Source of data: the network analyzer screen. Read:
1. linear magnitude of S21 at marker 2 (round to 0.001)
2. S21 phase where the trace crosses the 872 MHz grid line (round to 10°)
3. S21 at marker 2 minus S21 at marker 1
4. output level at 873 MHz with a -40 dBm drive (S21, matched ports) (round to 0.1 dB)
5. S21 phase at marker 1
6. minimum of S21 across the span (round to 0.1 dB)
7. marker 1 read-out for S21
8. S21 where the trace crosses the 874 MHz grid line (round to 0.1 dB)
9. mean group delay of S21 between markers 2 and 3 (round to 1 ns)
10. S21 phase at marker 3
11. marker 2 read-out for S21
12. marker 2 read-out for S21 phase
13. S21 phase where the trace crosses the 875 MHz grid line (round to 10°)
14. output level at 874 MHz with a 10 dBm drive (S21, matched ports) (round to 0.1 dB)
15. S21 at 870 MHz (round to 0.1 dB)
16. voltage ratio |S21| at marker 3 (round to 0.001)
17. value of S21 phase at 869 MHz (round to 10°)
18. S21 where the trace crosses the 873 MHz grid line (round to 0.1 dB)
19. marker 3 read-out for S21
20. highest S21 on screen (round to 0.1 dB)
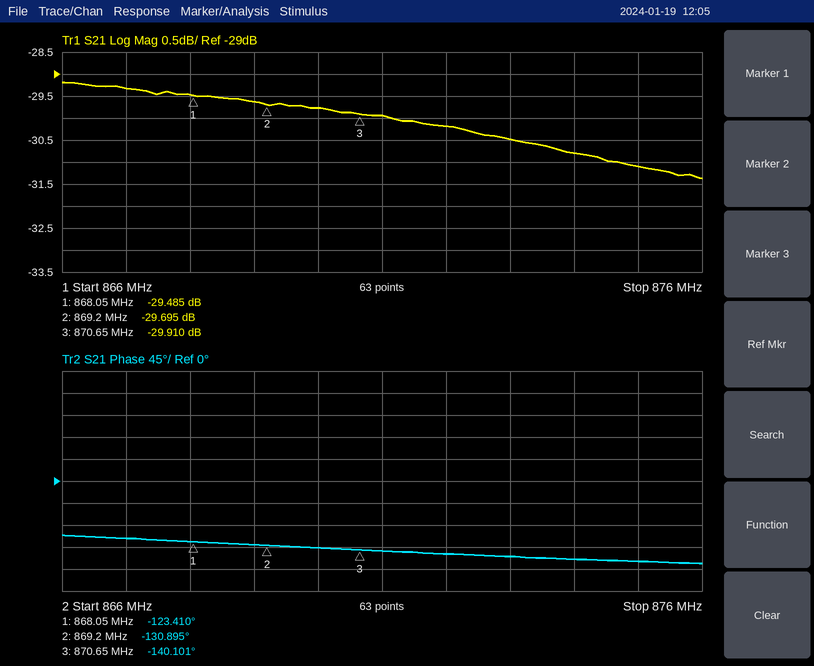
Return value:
0.033
-150°
-0.210 dB
-70.5 dBm
-123.410°
-31.4 dB
-29.485 dB
-30.8 dB
18 ns
-140.101°
-29.695 dB
-130.895°
-160°
-20.8 dBm
-29.8 dB
0.032
-130°
-30.5 dB
-29.910 dB
-29.2 dB
